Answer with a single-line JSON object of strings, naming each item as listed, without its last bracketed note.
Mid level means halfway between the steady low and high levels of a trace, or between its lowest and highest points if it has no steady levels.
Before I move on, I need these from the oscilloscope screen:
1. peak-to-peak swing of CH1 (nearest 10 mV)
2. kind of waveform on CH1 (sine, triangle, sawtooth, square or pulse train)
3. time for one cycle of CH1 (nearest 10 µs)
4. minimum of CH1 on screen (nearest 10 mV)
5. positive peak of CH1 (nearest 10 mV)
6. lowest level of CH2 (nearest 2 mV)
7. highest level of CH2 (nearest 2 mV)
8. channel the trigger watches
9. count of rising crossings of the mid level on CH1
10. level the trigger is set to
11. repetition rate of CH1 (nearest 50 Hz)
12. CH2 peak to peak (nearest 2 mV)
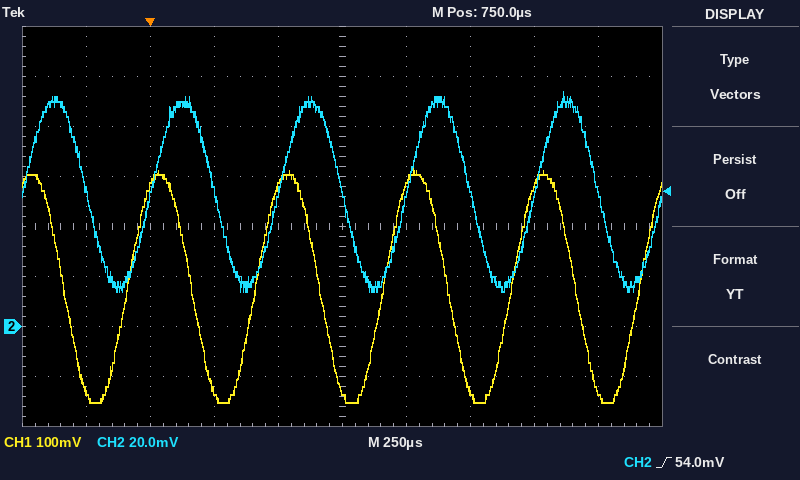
{"peak-to-peak swing of CH1": "470 mV", "kind of waveform on CH1": "sine", "time for one cycle of CH1": "500 µs", "minimum of CH1 on screen": "-150 mV", "positive peak of CH1": "320 mV", "lowest level of CH2": "14 mV", "highest level of CH2": "94 mV", "channel the trigger watches": "CH2", "count of rising crossings of the mid level on CH1": "5", "level the trigger is set to": "54.0 mV", "repetition rate of CH1": "2.00 kHz", "CH2 peak to peak": "80 mV"}
